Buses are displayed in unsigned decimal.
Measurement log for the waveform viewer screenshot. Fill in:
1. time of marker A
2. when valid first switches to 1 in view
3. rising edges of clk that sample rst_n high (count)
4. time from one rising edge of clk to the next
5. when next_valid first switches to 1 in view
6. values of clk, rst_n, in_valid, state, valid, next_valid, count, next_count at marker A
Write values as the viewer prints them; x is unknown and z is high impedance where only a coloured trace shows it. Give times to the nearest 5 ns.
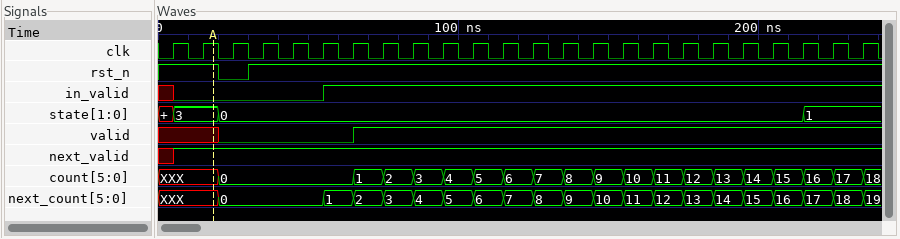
20 ns
65 ns
23
10 ns
5 ns
clk=1, rst_n=1, in_valid=0, state=3, valid=x, next_valid=1, count=XXX, next_count=XXX
